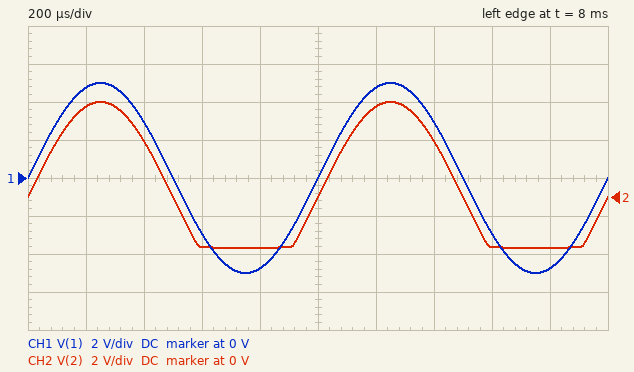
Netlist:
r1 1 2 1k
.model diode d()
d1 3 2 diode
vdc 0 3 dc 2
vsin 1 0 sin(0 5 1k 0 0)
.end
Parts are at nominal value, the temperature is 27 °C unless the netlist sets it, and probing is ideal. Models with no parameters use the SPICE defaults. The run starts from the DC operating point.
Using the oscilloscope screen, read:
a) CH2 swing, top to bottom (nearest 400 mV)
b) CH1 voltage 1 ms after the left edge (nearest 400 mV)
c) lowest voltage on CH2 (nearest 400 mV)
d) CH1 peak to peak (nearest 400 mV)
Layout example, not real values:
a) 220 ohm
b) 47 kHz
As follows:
a) 7.6 V
b) 0 V
c) -2.8 V
d) 10.0 V
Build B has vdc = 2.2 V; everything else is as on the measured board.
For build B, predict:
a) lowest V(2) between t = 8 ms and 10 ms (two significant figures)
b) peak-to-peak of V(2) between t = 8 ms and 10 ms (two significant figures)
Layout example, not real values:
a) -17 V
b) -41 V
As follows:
a) -2.9 V
b) 7.9 V
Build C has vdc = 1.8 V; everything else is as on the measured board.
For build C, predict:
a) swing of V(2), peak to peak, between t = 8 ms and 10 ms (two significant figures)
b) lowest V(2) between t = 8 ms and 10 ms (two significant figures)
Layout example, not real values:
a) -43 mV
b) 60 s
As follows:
a) 7.5 V
b) -2.5 V
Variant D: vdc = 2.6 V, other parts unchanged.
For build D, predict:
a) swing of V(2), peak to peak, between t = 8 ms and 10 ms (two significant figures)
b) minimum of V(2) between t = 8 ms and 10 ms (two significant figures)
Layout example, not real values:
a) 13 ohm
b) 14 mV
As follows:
a) 8.3 V
b) -3.3 V
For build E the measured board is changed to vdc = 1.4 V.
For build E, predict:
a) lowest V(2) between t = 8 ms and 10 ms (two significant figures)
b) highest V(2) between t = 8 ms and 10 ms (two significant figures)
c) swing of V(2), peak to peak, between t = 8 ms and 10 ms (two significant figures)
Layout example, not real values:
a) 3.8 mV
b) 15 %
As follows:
a) -2.1 V
b) 5.0 V
c) 7.1 V
